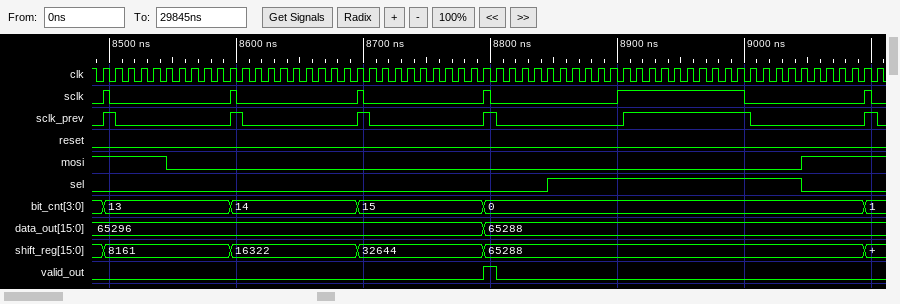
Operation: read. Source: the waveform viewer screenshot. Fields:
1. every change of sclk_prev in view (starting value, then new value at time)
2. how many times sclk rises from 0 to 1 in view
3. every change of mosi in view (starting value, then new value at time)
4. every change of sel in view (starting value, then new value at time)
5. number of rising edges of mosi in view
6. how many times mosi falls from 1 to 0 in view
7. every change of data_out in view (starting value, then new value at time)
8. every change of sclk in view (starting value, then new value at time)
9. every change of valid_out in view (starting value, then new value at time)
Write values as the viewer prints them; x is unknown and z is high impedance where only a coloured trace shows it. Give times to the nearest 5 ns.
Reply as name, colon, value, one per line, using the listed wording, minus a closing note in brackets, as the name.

every change of sclk_prev in view: 0, 1 at 8495 ns, 0 at 8505 ns, 1 at 8595 ns, 0 at 8605 ns, 1 at 8695 ns, 0 at 8705 ns, 1 at 8795 ns, 0 at 8805 ns, 1 at 8905 ns, 0 at 9005 ns, 1 at 9095 ns, 0 at 9105 ns
how many times sclk rises from 0 to 1 in view: 6
every change of mosi in view: 1, 0 at 8545 ns, 1 at 9045 ns
every change of sel in view: 0, 1 at 8845 ns, 0 at 9045 ns
number of rising edges of mosi in view: 1
how many times mosi falls from 1 to 0 in view: 1
every change of data_out in view: 65296, 65288 at 8795 ns
every change of sclk in view: 0, 1 at 8495 ns, 0 at 8500 ns, 1 at 8595 ns, 0 at 8600 ns, 1 at 8695 ns, 0 at 8700 ns, 1 at 8795 ns, 0 at 8800 ns, 1 at 8900 ns, 0 at 9000 ns, 1 at 9095 ns, 0 at 9100 ns
every change of valid_out in view: 0, 1 at 8795 ns, 0 at 8805 ns
